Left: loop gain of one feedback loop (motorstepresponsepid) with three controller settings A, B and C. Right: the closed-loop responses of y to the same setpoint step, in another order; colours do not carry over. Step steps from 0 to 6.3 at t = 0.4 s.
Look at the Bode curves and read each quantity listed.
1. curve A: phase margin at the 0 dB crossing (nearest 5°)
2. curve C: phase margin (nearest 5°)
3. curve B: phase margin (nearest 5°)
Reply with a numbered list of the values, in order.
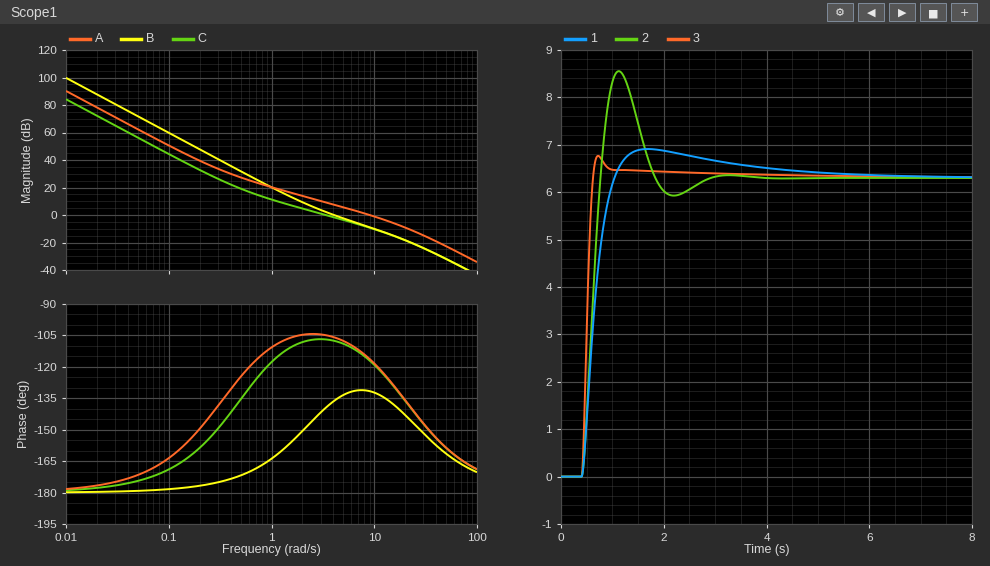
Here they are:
1. 65°
2. 75°
3. 45°
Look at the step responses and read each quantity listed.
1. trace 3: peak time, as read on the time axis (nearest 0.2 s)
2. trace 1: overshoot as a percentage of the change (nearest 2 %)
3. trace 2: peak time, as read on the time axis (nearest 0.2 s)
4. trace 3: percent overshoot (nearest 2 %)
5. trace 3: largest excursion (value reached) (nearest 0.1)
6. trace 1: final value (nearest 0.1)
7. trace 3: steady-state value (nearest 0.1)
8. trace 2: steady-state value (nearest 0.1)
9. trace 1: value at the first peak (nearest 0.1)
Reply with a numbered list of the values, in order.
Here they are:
1. 0.8 s
2. 10 %
3. 1.2 s
4. 8 %
5. 6.8
6. 6.3
7. 6.3
8. 6.3
9. 6.9
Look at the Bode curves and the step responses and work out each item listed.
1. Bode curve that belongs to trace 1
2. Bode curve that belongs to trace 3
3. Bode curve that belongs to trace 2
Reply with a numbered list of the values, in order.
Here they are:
1. C
2. A
3. B
